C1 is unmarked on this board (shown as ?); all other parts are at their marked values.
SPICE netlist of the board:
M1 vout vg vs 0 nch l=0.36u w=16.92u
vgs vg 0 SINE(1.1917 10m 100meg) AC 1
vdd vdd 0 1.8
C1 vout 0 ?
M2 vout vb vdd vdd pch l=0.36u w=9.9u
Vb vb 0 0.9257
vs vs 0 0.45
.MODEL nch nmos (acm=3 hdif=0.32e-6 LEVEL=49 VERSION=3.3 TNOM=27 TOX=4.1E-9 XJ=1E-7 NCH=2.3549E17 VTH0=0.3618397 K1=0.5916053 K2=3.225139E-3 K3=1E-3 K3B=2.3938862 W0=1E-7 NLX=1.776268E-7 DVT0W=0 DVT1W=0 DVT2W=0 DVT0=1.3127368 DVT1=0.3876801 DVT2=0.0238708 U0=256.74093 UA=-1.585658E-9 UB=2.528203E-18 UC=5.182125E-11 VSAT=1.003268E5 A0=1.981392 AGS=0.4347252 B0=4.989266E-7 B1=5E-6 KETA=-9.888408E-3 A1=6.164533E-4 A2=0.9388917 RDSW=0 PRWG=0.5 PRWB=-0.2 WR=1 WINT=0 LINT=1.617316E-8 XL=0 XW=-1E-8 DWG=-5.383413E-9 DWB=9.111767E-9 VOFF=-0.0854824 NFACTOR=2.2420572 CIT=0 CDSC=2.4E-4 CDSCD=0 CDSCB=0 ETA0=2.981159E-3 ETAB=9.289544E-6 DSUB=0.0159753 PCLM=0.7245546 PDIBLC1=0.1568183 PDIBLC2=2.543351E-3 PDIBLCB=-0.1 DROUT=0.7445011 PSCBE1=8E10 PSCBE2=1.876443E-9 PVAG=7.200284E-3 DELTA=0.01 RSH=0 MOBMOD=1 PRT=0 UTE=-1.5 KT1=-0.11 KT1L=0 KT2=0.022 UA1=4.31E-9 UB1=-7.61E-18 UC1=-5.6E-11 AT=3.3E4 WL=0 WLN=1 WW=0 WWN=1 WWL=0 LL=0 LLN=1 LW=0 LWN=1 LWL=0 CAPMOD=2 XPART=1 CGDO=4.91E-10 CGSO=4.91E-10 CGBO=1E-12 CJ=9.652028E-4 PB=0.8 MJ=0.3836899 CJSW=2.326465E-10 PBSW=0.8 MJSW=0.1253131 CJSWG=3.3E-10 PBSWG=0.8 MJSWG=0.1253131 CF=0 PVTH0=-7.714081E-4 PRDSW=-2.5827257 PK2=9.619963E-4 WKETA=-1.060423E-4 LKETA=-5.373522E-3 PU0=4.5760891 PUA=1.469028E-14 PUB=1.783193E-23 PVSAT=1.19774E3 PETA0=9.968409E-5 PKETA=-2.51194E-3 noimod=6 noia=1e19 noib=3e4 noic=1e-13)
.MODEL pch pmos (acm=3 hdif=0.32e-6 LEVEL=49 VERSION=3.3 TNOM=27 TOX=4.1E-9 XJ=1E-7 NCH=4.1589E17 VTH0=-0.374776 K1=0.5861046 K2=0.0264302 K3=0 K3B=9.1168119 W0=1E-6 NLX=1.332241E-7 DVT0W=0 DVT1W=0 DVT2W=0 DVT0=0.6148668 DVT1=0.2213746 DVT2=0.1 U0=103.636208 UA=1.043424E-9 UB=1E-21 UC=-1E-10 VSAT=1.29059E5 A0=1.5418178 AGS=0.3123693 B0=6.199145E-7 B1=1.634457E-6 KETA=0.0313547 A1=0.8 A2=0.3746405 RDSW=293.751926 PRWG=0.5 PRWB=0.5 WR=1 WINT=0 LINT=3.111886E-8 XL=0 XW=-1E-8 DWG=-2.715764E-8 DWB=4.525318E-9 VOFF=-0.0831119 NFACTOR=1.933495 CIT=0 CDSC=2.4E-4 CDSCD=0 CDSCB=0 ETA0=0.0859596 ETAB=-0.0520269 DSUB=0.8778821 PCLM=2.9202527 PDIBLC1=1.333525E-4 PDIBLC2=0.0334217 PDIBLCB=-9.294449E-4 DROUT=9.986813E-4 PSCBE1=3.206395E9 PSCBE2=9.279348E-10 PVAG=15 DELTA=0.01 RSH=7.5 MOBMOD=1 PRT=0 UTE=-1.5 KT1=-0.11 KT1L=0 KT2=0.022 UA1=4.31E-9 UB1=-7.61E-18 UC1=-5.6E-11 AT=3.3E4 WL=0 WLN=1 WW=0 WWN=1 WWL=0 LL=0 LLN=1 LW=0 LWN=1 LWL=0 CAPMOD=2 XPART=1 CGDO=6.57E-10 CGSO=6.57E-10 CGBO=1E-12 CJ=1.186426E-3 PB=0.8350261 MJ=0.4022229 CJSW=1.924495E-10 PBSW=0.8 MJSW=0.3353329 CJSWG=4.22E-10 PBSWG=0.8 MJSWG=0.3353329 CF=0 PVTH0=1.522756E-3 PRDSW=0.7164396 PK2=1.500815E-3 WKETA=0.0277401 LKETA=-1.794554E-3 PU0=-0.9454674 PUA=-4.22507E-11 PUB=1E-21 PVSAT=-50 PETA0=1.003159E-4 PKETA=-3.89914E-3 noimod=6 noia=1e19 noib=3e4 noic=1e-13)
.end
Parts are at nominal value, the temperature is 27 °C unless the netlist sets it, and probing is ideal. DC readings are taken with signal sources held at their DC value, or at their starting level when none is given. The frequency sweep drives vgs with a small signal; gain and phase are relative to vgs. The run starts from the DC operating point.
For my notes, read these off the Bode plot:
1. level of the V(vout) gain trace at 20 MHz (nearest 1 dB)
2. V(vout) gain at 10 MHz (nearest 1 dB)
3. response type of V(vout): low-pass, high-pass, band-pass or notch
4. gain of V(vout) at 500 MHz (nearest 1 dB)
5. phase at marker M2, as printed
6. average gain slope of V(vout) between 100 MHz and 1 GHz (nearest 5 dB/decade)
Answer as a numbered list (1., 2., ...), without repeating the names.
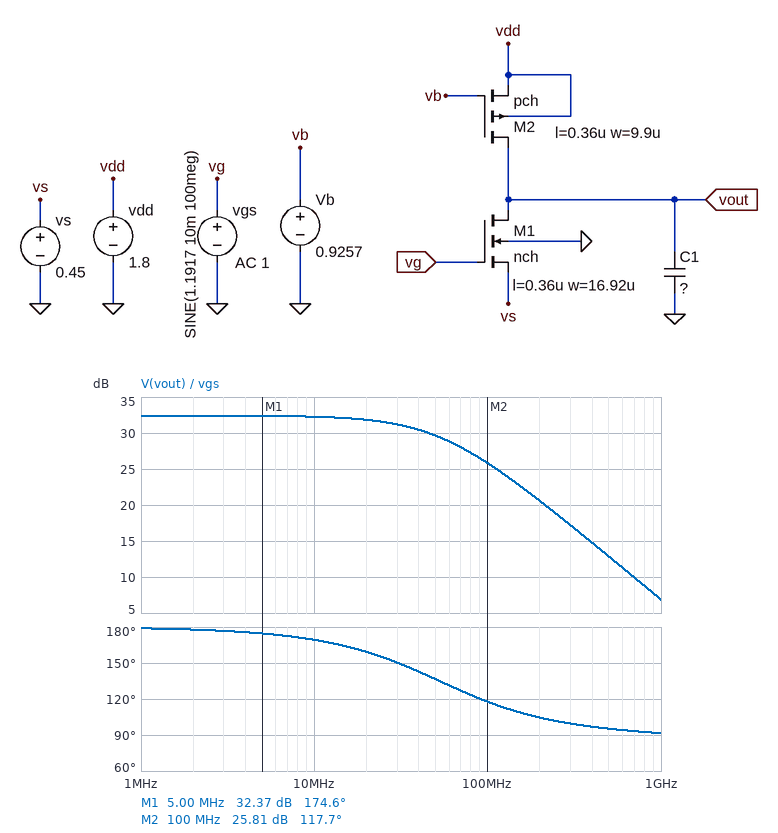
1. 32 dB
2. 32 dB
3. low-pass
4. 13 dB
5. 117.7 deg
6. -20 dB/decade
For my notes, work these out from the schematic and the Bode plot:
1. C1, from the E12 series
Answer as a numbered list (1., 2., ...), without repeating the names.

1. 100 fF
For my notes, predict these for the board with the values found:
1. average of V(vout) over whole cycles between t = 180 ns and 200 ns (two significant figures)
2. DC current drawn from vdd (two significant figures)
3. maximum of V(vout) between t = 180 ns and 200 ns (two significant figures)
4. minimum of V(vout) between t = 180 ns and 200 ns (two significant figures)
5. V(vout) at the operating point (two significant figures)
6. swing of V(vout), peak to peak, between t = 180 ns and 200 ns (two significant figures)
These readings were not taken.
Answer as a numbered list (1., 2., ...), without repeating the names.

1. 1.1 V
2. 170 µA
3. 1.3 V
4. 900 mV
5. 1.1 V
6. 390 mV
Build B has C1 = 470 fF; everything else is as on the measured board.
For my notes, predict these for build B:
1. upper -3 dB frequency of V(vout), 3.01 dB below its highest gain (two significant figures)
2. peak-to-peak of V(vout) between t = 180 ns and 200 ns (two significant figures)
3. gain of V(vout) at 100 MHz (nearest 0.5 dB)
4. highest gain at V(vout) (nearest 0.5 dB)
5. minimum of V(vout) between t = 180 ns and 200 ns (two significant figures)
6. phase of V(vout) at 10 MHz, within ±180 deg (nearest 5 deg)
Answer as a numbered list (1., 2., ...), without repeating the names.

1. 15 MHz
2. 120 mV
3. 15.5 dB
4. 32.5 dB
5. 1.0 V
6. 145 deg
